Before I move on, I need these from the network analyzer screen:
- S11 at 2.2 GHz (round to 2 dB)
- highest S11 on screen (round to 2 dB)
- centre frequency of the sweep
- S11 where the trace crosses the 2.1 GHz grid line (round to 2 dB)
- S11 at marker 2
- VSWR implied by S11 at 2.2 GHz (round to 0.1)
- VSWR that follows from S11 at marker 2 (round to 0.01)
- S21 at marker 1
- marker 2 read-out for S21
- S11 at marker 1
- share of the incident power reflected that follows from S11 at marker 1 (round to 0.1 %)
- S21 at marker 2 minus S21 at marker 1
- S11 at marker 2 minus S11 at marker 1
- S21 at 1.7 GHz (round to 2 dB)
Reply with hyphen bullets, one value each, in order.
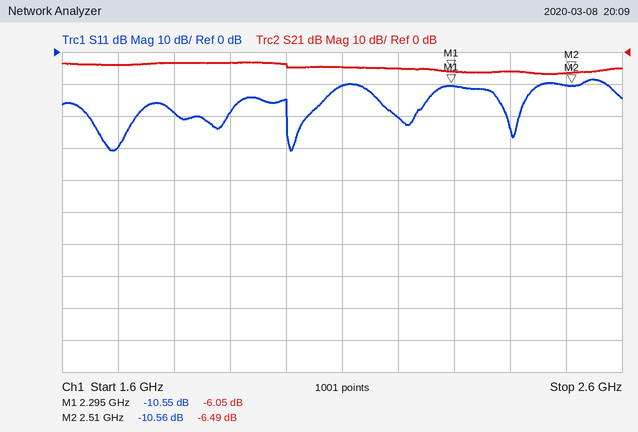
- -20 dB
- -8 dB
- 2.1 GHz
- -10 dB
- -10.56 dB
- 1.2
- 1.84
- -6.05 dB
- -6.49 dB
- -10.55 dB
- 8.8 %
- -0.44 dB
- -0.01 dB
- -4 dB
